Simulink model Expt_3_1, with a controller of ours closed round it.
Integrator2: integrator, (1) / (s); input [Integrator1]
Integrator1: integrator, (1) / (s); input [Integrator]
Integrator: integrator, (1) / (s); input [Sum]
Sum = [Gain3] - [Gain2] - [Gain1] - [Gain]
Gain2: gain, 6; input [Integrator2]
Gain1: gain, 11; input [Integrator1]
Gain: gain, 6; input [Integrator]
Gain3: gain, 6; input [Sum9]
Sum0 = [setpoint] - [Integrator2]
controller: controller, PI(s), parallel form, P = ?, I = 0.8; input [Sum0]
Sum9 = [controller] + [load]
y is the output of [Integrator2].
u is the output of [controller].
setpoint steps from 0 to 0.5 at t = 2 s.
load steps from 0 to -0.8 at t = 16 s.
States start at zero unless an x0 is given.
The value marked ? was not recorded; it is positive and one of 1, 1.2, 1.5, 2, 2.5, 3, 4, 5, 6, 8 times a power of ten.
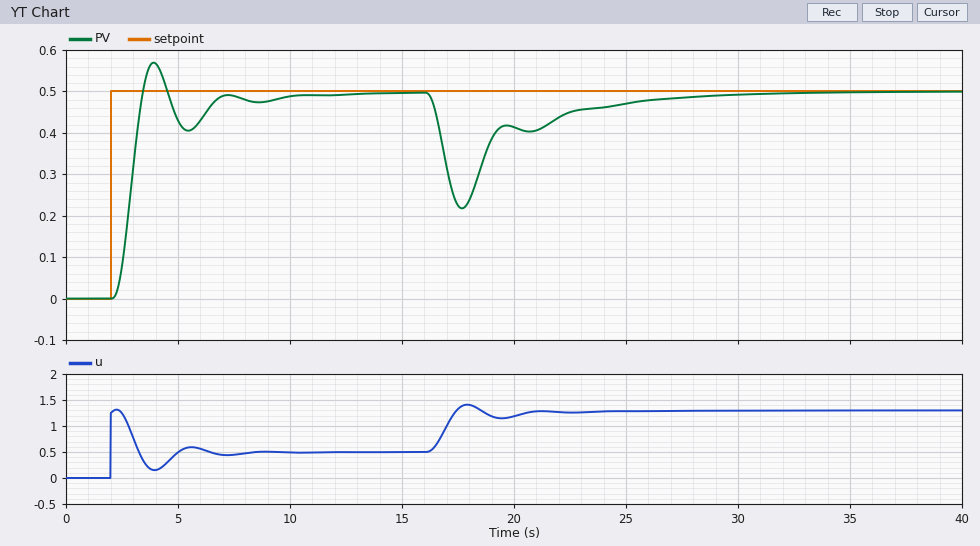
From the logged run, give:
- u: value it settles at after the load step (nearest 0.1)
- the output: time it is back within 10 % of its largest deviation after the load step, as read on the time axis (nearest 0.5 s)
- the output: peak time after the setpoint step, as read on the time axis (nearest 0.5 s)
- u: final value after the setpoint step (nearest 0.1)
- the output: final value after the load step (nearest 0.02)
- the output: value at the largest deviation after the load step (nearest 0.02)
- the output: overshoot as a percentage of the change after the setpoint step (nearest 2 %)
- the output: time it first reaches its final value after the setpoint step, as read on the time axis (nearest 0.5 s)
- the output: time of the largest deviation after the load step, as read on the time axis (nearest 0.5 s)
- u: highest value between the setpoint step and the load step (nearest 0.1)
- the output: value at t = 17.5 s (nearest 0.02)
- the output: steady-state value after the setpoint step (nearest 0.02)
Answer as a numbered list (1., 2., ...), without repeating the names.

1. 1.3
2. 25.0 s
3. 4.0 s
4. 0.5
5. 0.50
6. 0.22
7. 14 %
8. 3.5 s
9. 17.5 s
10. 1.3
11. 0.22
12. 0.50
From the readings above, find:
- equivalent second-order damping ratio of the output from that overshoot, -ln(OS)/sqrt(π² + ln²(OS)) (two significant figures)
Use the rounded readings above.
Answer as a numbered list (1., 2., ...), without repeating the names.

1. 0.53
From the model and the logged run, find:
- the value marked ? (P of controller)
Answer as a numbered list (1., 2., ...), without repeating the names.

1. 2.5
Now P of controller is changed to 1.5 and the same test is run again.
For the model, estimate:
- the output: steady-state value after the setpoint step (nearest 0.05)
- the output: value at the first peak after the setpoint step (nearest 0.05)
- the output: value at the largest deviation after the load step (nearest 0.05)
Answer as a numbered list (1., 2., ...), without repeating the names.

1. 0.50
2. 0.55
3. 0.15
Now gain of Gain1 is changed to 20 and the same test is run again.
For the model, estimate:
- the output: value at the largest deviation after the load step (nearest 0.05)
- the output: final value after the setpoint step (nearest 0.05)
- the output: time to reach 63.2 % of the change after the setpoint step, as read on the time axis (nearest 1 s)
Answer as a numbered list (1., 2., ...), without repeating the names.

1. 0.30
2. 0.50
3. 3 s
